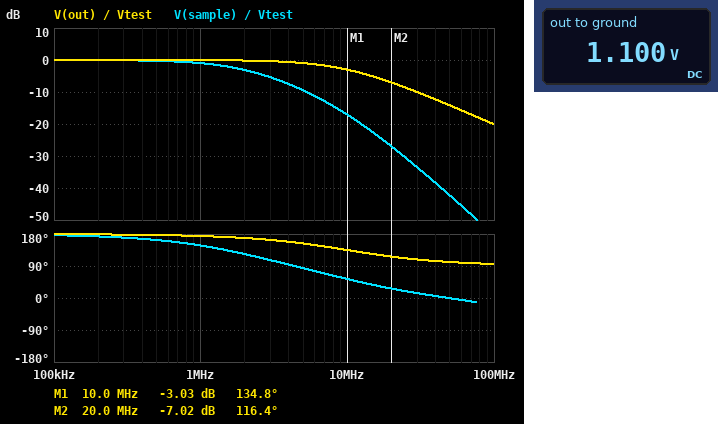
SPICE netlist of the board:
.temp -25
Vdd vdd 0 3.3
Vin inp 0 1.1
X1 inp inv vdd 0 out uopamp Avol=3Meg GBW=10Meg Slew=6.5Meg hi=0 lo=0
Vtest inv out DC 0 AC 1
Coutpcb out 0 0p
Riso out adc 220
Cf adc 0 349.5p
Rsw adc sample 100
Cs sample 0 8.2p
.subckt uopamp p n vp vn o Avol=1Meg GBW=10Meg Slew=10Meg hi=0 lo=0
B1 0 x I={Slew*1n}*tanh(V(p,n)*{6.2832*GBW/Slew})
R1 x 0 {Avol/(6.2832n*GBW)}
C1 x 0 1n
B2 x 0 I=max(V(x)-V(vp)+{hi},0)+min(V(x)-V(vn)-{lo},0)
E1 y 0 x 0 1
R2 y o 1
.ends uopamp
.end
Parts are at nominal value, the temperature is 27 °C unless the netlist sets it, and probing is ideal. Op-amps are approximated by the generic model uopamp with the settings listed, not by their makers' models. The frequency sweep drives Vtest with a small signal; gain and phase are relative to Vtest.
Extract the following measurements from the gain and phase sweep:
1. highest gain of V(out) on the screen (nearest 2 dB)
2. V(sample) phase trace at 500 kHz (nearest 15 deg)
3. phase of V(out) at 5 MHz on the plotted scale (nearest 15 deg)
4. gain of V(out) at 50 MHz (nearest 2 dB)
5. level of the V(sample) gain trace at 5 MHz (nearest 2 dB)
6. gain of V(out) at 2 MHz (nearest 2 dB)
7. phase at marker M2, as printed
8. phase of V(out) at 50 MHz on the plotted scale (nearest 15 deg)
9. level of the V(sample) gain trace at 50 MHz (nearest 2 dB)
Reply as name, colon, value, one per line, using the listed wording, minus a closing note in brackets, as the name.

highest gain of V(out) on the screen: 0 dB
V(sample) phase trace at 500 kHz: 165 deg
phase of V(out) at 5 MHz on the plotted scale: 150 deg
gain of V(out) at 50 MHz: -14 dB
level of the V(sample) gain trace at 5 MHz: -10 dB
gain of V(out) at 2 MHz: 0 dB
phase at marker M2, as printed: 116.4 deg
phase of V(out) at 50 MHz on the plotted scale: 105 deg
level of the V(sample) gain trace at 50 MHz: -42 dB
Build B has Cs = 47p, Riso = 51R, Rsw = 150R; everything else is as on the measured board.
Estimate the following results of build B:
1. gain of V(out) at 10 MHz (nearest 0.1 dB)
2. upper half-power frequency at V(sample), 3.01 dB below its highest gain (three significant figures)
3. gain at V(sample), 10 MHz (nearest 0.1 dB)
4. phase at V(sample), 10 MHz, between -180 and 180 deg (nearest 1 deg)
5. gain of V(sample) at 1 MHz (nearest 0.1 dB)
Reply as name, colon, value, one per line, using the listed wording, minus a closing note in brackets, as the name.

gain of V(out) at 10 MHz: -3.0 dB
upper half-power frequency at V(sample), 3.01 dB below its highest gain: 5.31 MHz
gain at V(sample), 10 MHz: -8.1 dB
phase at V(sample), 10 MHz, between -180 and 180 deg: 61 deg
gain of V(sample) at 1 MHz: -0.1 dB
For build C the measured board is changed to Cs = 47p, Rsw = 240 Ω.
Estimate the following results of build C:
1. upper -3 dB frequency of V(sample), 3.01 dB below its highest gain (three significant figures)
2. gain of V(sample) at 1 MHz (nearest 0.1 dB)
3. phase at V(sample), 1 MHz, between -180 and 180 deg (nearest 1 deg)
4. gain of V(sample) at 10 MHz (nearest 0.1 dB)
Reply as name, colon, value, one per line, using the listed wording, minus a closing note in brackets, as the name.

upper -3 dB frequency of V(sample), 3.01 dB below its highest gain: 1.72 MHz
gain of V(sample) at 1 MHz: -1.2 dB
phase at V(sample), 1 MHz, between -180 and 180 deg: 142 deg
gain of V(sample) at 10 MHz: -19.5 dB
